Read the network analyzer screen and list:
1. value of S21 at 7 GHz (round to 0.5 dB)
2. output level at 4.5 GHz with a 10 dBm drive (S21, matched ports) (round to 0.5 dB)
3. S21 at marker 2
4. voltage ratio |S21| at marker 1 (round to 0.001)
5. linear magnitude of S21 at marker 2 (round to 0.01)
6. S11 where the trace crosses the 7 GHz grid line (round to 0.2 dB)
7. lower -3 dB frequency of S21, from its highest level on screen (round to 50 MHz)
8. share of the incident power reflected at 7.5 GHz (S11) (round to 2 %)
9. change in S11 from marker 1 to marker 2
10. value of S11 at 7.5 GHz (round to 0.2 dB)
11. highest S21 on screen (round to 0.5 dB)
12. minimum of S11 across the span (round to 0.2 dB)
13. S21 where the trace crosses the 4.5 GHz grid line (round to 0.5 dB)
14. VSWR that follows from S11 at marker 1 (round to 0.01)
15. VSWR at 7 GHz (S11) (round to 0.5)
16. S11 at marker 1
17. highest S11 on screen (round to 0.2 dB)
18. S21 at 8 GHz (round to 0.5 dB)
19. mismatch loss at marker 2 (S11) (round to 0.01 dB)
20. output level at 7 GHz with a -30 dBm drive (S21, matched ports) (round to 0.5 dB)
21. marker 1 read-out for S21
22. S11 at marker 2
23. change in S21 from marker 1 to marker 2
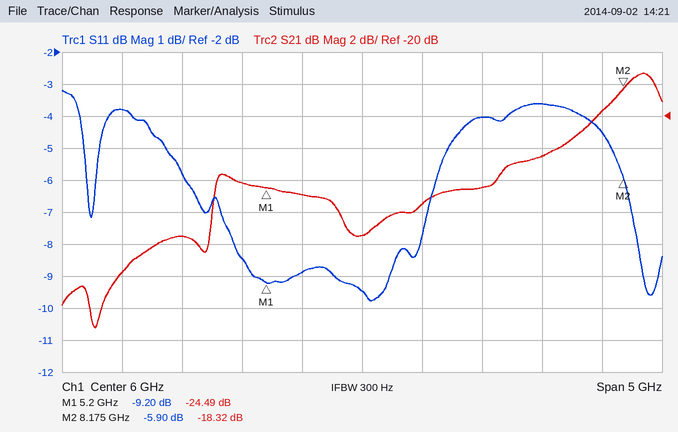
-24.5 dB
-17.5 dBm
-18.32 dB
0.060
0.12
-4.0 dB
7.90 GHz
44 %
3.30 dB
-3.6 dB
-17.5 dB
-9.8 dB
-27.5 dB
2.06
4.5
-9.20 dB
-3.2 dB
-19.5 dB
1.29 dB
-54.5 dBm
-24.49 dB
-5.90 dB
6.17 dB
